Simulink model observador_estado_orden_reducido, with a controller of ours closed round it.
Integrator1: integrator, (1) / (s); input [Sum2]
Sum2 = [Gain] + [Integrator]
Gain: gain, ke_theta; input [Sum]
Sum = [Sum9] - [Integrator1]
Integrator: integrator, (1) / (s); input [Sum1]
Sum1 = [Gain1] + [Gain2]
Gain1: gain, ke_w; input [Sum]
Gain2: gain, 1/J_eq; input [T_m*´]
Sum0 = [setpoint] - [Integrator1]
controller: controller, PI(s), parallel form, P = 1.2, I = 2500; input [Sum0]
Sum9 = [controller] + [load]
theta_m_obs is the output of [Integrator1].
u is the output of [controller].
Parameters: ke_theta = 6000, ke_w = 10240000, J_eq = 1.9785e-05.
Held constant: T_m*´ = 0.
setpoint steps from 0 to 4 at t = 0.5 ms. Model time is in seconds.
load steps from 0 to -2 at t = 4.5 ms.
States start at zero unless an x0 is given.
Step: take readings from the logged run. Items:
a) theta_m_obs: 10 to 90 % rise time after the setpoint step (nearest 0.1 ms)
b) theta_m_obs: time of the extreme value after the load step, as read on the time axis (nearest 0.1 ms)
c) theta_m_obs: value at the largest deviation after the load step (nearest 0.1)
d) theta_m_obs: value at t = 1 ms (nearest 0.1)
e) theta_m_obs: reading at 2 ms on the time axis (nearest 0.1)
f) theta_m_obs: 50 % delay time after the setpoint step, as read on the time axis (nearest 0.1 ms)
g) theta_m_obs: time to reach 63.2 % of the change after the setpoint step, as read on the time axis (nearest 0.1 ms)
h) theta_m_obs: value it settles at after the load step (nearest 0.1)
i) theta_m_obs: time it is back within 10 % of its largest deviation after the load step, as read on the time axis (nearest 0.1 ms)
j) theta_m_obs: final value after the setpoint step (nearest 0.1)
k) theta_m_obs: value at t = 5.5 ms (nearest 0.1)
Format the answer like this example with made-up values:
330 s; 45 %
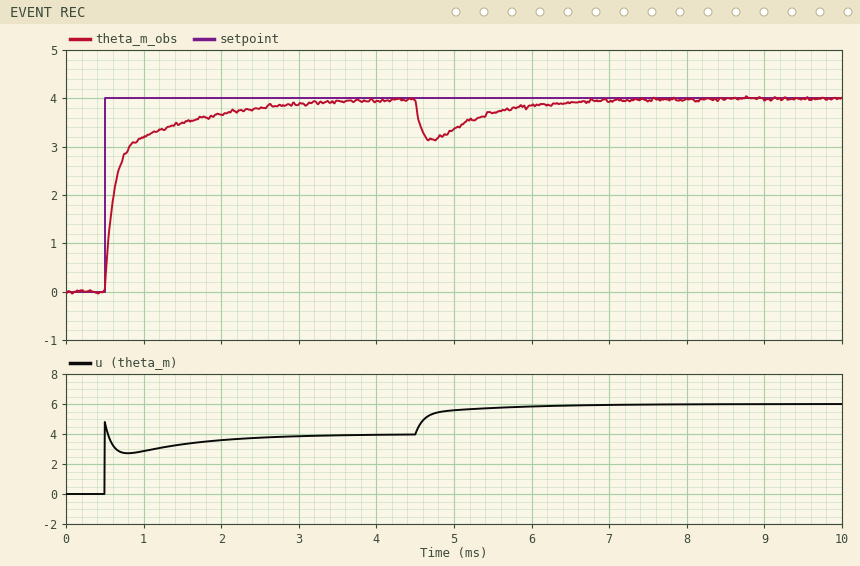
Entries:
1.2 ms; 4.7 ms; 3.1; 3.2; 3.7; 0.6 ms; 0.7 ms; 4.0; 6.5 ms; 4.0; 3.7
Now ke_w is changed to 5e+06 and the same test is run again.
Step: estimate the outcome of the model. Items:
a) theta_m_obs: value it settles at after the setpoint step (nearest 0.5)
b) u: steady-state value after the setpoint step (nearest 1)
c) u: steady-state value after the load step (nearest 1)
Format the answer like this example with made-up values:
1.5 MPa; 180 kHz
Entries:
4.0; 4; 6
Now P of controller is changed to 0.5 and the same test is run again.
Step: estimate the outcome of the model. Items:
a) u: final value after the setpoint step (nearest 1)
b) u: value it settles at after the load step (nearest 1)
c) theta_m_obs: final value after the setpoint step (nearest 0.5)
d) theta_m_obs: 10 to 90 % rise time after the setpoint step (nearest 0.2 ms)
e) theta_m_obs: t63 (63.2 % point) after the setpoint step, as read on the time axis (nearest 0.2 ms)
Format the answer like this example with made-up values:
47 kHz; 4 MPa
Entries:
4; 6; 4.0; 0.8 ms; 0.8 ms
